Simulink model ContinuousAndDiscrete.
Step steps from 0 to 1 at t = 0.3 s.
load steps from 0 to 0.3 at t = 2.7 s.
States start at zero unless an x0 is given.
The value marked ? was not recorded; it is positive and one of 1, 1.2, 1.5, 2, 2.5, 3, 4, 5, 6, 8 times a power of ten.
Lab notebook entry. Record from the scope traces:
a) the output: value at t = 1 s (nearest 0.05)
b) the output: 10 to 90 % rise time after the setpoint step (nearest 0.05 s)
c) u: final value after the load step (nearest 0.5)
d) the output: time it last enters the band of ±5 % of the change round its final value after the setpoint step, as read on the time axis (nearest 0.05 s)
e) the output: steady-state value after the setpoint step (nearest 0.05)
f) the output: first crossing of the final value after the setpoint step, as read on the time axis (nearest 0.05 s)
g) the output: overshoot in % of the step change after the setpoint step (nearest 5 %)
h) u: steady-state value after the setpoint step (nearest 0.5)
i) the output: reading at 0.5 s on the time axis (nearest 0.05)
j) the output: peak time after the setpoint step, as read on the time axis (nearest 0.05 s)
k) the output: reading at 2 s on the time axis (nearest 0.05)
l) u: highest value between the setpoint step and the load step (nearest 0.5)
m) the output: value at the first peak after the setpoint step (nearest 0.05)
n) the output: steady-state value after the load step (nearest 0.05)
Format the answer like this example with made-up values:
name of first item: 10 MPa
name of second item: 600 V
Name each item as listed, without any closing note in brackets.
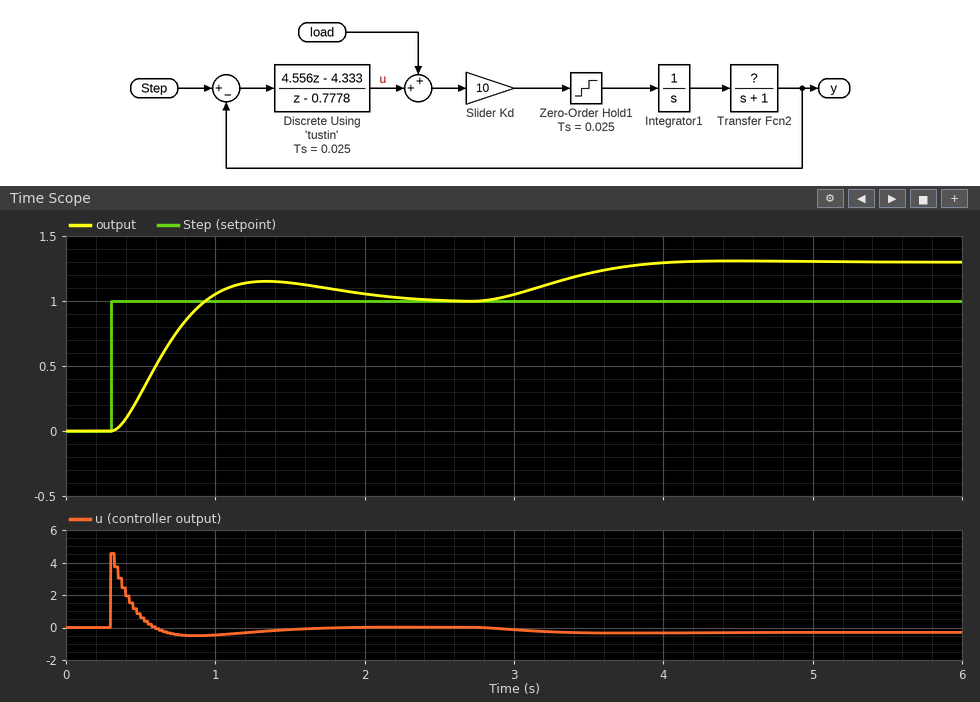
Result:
the output: value at t = 1 s: 1.05
the output: 10 to 90 % rise time after the setpoint step: 0.45 s
u: final value after the load step: -0.5
the output: time it last enters the band of ±5 % of the change round its final value after the setpoint step, as read on the time axis: 2.05 s
the output: steady-state value after the setpoint step: 1.00
the output: first crossing of the final value after the setpoint step, as read on the time axis: 0.95 s
the output: overshoot in % of the step change after the setpoint step: 15 %
u: steady-state value after the setpoint step: 0.0
the output: reading at 0.5 s on the time axis: 0.30
the output: peak time after the setpoint step, as read on the time axis: 1.35 s
the output: reading at 2 s on the time axis: 1.05
u: highest value between the setpoint step and the load step: 4.5
the output: value at the first peak after the setpoint step: 1.15
the output: steady-state value after the load step: 1.30
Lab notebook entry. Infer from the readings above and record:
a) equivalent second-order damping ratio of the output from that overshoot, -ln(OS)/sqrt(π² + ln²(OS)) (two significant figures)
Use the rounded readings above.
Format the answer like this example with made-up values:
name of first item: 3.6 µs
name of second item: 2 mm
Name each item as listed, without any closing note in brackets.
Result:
equivalent second-order damping ratio of the output from that overshoot, -ln(OS)/sqrt(π² + ln²(OS)): 0.52
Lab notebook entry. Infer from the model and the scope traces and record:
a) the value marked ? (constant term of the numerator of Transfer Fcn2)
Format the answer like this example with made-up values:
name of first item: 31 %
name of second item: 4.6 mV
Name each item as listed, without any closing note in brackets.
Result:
the value marked ?: 0.5
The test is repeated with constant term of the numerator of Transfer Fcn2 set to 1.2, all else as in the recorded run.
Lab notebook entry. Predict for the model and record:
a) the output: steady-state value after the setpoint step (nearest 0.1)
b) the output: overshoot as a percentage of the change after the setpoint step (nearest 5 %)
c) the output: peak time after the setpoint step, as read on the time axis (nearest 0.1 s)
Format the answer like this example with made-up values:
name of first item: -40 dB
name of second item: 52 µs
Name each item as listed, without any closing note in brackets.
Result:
the output: steady-state value after the setpoint step: 1.0
the output: overshoot as a percentage of the change after the setpoint step: 25 %
the output: peak time after the setpoint step, as read on the time axis: 0.8 s
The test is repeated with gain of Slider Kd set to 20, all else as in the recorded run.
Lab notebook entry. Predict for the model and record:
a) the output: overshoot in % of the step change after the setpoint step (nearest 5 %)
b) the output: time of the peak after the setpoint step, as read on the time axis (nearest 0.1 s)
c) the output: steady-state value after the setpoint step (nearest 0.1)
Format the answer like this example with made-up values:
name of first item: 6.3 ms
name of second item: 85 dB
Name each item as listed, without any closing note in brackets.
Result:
the output: overshoot in % of the step change after the setpoint step: 20 %
the output: time of the peak after the setpoint step, as read on the time axis: 0.9 s
the output: steady-state value after the setpoint step: 1.0
